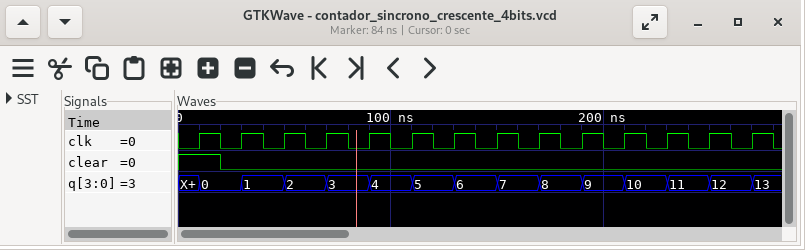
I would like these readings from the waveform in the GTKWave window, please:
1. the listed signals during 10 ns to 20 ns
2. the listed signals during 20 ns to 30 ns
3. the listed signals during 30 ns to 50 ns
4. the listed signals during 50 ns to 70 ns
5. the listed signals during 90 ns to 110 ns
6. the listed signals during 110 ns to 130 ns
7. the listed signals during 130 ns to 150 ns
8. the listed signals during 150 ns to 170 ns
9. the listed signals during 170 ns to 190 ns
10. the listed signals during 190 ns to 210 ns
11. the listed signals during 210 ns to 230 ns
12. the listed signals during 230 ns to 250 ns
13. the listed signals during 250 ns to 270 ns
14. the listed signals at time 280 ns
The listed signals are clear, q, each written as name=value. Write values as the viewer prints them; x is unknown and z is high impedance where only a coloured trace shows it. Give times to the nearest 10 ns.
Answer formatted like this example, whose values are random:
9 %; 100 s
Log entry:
clear=1, q=0; clear=0, q=0; clear=0, q=1; clear=0, q=2; clear=0, q=4; clear=0, q=5; clear=0, q=6; clear=0, q=7; clear=0, q=8; clear=0, q=9; clear=0, q=10; clear=0, q=11; clear=0, q=12; clear=0, q=13
